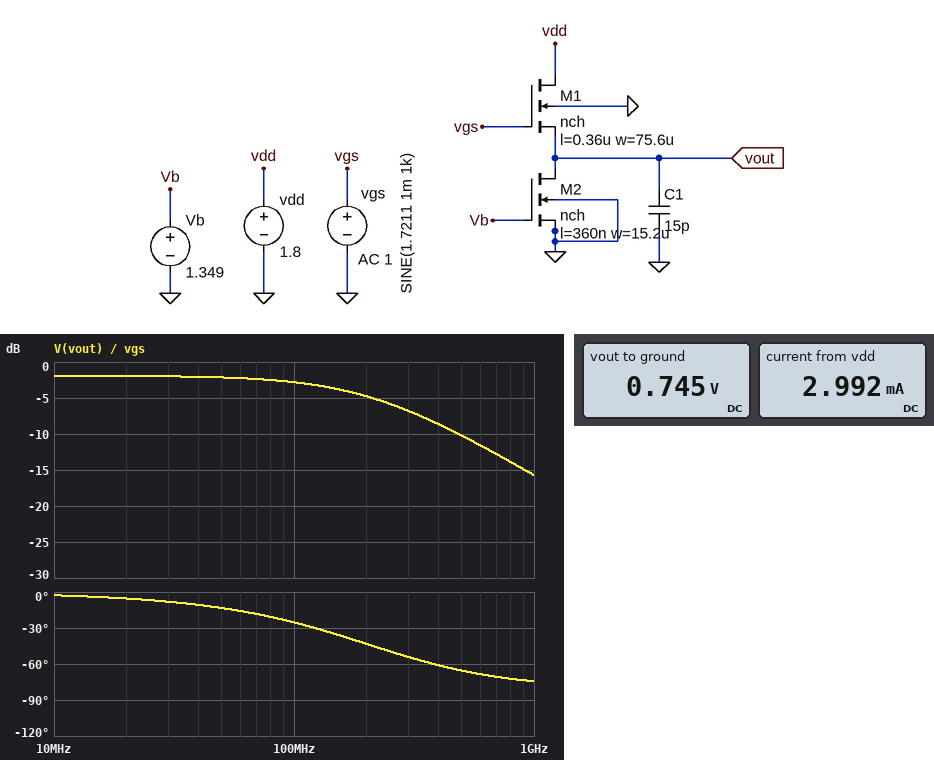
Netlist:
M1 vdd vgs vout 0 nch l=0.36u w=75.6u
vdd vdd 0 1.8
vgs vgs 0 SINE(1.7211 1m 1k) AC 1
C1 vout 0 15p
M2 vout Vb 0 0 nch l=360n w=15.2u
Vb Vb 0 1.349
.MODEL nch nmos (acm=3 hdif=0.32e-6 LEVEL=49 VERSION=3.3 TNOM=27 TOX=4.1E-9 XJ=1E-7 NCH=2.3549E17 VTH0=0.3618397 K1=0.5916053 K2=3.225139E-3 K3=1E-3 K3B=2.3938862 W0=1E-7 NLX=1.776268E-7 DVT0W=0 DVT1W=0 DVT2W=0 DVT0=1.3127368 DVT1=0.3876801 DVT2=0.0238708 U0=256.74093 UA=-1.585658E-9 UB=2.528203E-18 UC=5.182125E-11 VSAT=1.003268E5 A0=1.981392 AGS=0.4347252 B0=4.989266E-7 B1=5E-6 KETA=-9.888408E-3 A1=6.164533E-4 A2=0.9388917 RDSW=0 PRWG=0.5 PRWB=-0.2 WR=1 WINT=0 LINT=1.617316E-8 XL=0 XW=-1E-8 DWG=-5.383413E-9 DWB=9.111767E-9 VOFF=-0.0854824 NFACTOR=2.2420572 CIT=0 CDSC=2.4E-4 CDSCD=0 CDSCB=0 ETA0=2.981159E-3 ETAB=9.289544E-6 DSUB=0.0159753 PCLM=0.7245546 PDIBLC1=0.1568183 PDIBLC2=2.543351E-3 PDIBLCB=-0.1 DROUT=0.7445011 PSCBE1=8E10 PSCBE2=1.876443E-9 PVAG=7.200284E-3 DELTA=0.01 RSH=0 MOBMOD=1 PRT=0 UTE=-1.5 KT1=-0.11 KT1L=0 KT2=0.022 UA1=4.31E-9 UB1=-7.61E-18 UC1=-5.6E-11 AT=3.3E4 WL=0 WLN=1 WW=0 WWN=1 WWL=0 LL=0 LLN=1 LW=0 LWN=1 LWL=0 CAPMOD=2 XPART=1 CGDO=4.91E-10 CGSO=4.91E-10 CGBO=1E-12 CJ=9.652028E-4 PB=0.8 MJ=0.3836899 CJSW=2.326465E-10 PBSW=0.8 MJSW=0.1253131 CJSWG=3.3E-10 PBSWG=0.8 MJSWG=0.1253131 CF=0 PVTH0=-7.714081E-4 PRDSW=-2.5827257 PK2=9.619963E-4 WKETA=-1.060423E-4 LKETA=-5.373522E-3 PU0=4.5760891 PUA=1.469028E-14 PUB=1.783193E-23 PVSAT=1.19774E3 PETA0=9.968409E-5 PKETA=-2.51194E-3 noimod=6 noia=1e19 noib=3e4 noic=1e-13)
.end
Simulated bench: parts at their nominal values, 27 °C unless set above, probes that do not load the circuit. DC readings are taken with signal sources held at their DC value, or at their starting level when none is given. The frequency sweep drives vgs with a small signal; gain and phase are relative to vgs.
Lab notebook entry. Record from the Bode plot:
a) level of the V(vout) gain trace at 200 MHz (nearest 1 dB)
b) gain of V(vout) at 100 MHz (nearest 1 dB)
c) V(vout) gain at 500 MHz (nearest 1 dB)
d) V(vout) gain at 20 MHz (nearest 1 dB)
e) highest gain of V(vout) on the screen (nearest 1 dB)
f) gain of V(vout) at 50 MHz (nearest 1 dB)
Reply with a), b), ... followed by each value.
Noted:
a) -5 dB
b) -3 dB
c) -10 dB
d) -2 dB
e) -2 dB
f) -2 dB
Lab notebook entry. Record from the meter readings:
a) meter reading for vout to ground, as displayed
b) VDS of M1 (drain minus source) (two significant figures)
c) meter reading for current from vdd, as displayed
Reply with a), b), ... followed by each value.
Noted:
a) 0.745 V
b) 1.1 V
c) 2.992 mA
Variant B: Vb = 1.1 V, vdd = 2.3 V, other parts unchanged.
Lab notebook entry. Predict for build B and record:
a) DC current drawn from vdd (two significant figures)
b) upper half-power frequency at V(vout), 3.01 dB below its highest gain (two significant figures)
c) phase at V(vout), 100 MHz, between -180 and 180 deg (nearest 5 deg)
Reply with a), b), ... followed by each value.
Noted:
a) 1.8 mA
b) 170 MHz
c) -30 deg
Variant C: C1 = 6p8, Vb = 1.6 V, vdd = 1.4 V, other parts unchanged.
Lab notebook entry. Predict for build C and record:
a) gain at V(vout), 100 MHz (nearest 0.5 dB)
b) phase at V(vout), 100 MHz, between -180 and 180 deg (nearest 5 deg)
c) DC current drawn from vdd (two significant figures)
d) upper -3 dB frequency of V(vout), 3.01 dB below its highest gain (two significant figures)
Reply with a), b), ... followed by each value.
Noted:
a) -2.5 dB
b) -10 deg
c) 4.3 mA
d) 520 MHz
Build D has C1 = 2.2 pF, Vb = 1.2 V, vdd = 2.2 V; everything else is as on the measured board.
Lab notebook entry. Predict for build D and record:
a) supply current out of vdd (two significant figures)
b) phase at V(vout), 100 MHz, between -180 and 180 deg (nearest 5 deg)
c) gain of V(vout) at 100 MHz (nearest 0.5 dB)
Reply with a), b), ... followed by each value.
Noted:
a) 2.2 mA
b) -5 deg
c) -2.0 dB
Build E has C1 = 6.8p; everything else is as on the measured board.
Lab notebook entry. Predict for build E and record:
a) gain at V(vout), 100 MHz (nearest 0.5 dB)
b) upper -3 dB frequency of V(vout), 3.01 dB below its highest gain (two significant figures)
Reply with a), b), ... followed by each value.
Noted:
a) -2.0 dB
b) 450 MHz
